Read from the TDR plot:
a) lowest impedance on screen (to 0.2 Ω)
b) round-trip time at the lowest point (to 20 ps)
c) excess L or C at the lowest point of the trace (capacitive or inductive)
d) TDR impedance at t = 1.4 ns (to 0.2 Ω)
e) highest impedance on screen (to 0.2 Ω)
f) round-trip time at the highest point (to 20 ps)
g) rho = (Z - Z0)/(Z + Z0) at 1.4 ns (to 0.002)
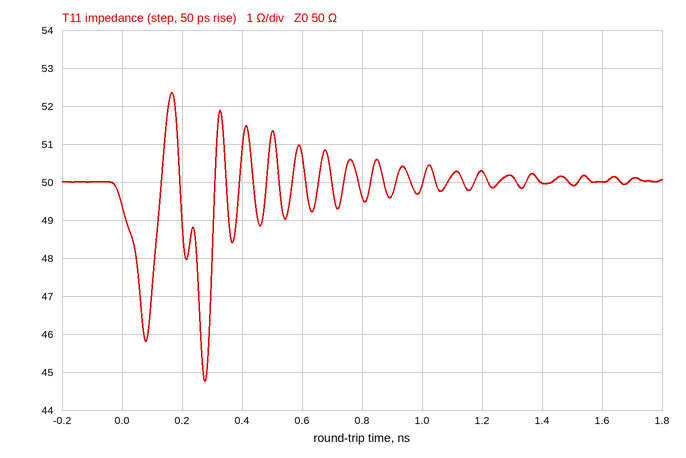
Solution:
44.8 Ω
280 ps
capacitive
50.0 Ω
52.4 Ω
160 ps
0.000
